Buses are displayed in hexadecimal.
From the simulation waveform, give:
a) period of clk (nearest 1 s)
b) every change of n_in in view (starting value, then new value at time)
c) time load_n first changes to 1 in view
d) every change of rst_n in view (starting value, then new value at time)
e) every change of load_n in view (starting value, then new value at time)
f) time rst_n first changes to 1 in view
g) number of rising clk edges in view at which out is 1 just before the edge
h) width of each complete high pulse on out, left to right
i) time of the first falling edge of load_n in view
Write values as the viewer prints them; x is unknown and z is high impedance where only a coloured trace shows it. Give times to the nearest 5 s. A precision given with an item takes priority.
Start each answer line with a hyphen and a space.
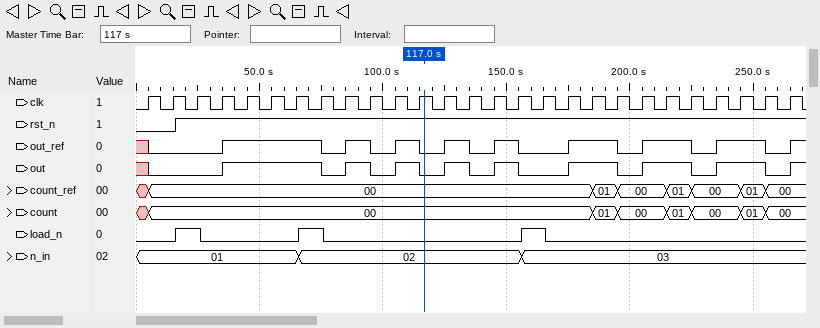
- 10 s
- 01, 02 at 65 s, 03 at 155 s
- 15 s
- 0, 1 at 15 s
- 0, 1 at 15 s, 0 at 25 s, 1 at 65 s, 0 at 75 s, 1 at 155 s, 0 at 165 s
- 15 s
- 14
- 40 s, 10 s, 10 s, 10 s, 10 s, 20 s, 20 s, 20 s
- 25 s
